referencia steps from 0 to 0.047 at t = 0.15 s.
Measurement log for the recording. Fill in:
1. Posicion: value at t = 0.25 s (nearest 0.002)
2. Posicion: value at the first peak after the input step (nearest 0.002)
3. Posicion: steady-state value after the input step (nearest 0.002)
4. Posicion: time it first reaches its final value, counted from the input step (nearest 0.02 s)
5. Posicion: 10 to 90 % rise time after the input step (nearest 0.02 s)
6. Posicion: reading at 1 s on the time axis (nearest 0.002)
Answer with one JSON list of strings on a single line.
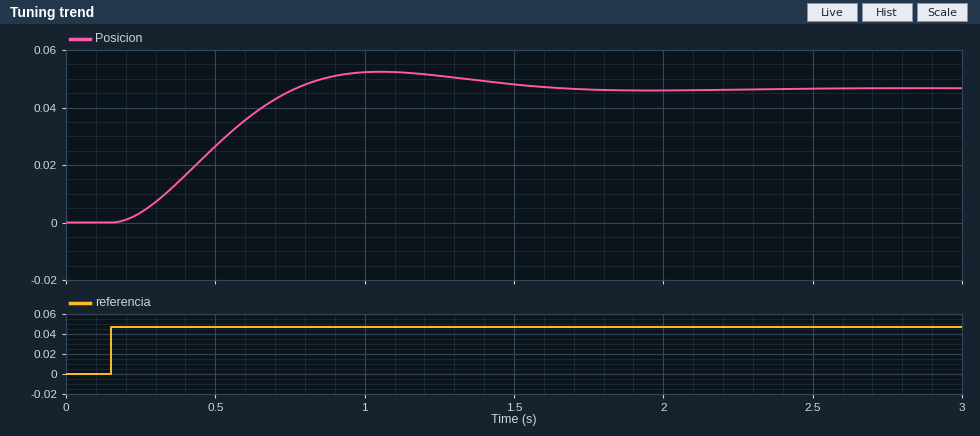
["0.004", "0.052", "0.046", "0.62 s", "0.42 s", "0.052"]
